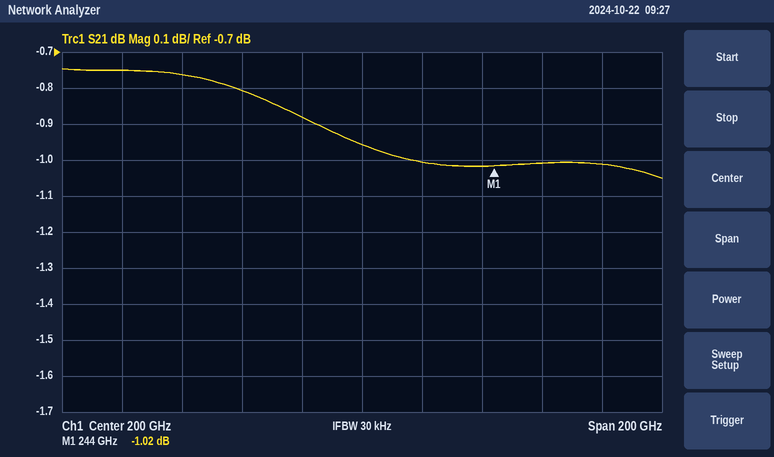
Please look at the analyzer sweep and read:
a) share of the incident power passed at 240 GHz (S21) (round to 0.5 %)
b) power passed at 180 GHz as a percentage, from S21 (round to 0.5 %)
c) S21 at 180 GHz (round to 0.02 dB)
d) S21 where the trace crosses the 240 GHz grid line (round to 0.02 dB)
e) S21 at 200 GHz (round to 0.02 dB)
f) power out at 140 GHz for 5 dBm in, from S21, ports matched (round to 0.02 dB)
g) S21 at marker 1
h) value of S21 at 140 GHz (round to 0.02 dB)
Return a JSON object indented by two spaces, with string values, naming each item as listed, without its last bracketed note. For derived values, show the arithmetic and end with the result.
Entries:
{
  "share of the incident power passed at 240 GHz (S21)": "10^(-1.02/10) ≈ 79.1 %, so 79.0 % to the nearest 0.5 %",
  "power passed at 180 GHz as a percentage, from S21": "10^(-0.88/10) ≈ 81.7 %, so 81.5 % to the nearest 0.5 %",
  "S21 at 180 GHz": "-0.88 dB",
  "S21 where the trace crosses the 240 GHz grid line": "-1.02 dB",
  "S21 at 200 GHz": "-0.96 dB",
  "power out at 140 GHz for 5 dBm in, from S21, ports matched": "5 dBm + (-0.76 dB) = 4.24 dBm",
  "S21 at marker 1": "-1.02 dB",
  "value of S21 at 140 GHz": "-0.76 dB"
}
